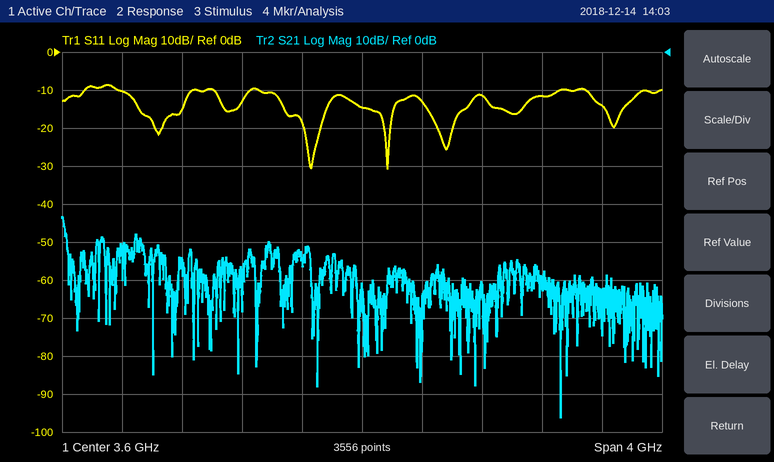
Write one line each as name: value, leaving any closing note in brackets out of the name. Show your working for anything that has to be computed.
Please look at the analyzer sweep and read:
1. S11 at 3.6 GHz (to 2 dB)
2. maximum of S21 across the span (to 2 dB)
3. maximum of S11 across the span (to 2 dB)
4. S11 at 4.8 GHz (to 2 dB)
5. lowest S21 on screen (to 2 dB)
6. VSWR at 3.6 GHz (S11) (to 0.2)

S11 at 3.6 GHz: -14 dB
maximum of S21 across the span: -44 dB
maximum of S11 across the span: -8 dB
S11 at 4.8 GHz: -12 dB
lowest S21 on screen: -96 dB
VSWR at 3.6 GHz (S11): |Γ| = 10^(-14/20) = 0.1995; VSWR = (1 + 0.1995)/(1 − 0.1995) ≈ 1.50, so 1.4 to the nearest 0.2
